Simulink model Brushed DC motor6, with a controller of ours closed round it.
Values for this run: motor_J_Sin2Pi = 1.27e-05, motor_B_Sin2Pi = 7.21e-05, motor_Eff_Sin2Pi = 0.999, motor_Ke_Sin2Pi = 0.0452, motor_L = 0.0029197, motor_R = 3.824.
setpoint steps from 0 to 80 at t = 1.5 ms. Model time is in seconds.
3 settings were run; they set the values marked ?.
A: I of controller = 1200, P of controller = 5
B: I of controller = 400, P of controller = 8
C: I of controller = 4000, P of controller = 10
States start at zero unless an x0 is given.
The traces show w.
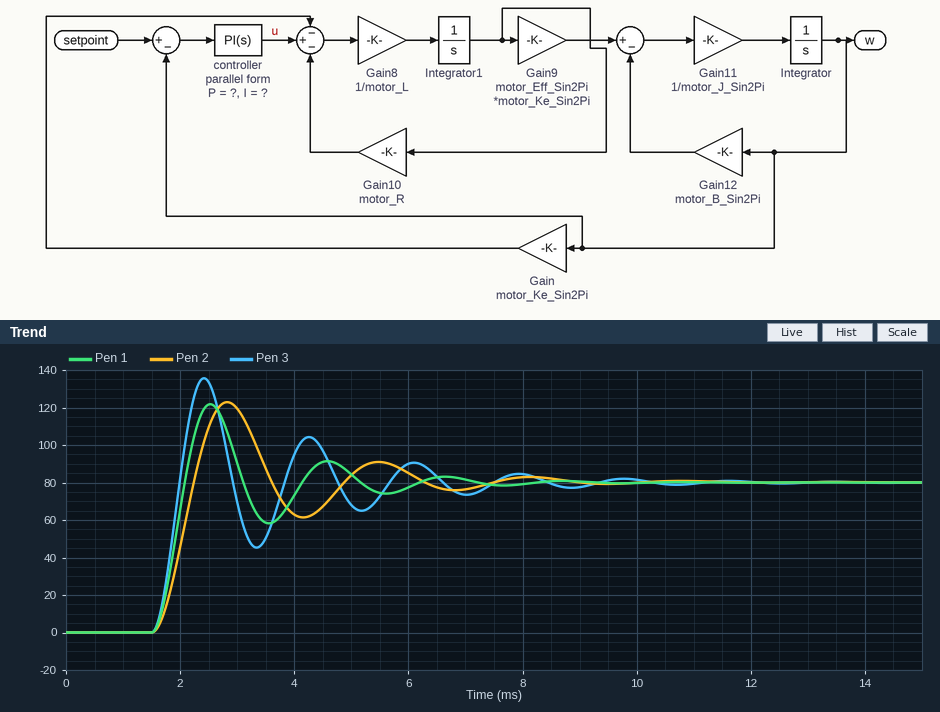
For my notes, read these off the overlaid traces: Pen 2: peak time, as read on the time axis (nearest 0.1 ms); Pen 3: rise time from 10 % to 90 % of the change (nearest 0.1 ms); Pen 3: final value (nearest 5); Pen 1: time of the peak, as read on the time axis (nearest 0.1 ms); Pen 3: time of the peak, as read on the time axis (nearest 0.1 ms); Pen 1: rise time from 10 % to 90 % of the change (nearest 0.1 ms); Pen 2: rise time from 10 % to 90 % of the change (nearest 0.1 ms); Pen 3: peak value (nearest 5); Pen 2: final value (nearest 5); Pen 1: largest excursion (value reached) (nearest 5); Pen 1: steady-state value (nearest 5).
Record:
2.8 ms
0.3 ms
80
2.5 ms
2.4 ms
0.4 ms
0.5 ms
135
80
120
80
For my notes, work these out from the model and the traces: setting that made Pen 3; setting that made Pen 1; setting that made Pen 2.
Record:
C
B
A
